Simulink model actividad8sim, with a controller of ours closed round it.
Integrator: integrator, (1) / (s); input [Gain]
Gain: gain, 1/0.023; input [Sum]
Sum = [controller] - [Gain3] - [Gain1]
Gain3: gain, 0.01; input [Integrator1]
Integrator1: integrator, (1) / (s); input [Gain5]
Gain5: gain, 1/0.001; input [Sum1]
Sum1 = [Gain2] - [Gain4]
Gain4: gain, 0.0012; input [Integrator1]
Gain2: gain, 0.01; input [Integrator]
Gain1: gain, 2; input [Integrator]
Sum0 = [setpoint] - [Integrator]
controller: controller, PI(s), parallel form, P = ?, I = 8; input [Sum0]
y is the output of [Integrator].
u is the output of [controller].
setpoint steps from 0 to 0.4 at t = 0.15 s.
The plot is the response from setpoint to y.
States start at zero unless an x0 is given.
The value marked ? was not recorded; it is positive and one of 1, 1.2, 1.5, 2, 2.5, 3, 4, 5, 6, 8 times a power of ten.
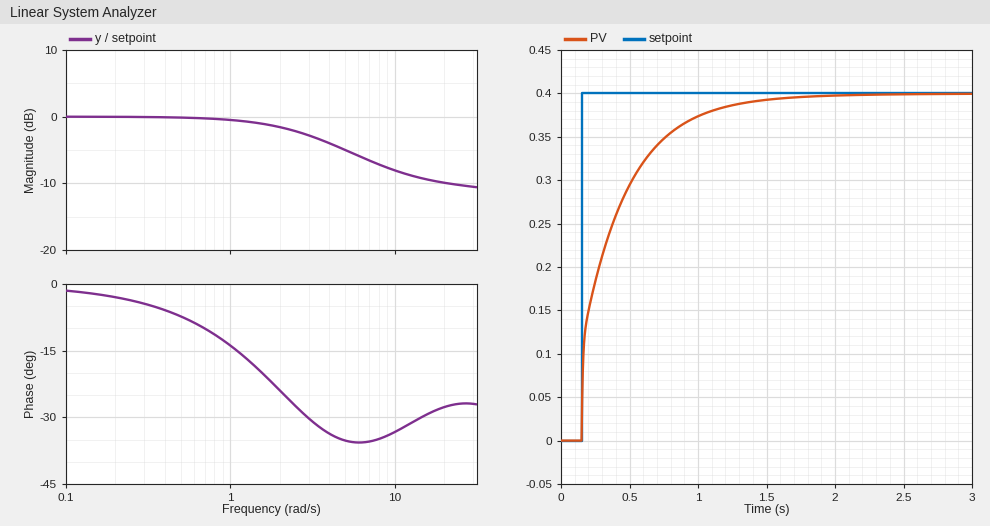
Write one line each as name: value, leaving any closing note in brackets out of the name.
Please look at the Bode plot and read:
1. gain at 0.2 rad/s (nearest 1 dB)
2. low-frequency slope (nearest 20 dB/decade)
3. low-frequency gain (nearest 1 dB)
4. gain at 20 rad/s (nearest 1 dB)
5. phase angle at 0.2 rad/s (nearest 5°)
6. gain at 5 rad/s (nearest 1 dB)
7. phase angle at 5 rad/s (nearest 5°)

gain at 0.2 rad/s: 0 dB
low-frequency slope: 0 dB/decade
low-frequency gain: 0 dB
gain at 20 rad/s: -10 dB
phase angle at 0.2 rad/s: -5°
gain at 5 rad/s: -5 dB
phase angle at 5 rad/s: -35°
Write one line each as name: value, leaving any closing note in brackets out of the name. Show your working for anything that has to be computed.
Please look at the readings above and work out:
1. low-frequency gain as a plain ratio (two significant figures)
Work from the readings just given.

low-frequency gain as a plain ratio: 10^(0 / 20) = 1.0
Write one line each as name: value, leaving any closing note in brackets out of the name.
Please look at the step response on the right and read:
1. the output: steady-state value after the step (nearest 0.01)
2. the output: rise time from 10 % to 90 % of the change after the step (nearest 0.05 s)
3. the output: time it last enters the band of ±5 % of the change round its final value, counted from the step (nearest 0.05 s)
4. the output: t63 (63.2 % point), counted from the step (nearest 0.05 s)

the output: steady-state value after the step: 0.40
the output: rise time from 10 % to 90 % of the change after the step: 0.70 s
the output: time it last enters the band of ±5 % of the change round its final value, counted from the step: 0.95 s
the output: t63 (63.2 % point), counted from the step: 0.25 s
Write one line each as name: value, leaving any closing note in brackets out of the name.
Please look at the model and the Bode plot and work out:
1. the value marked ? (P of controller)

the value marked ?: 0.8
